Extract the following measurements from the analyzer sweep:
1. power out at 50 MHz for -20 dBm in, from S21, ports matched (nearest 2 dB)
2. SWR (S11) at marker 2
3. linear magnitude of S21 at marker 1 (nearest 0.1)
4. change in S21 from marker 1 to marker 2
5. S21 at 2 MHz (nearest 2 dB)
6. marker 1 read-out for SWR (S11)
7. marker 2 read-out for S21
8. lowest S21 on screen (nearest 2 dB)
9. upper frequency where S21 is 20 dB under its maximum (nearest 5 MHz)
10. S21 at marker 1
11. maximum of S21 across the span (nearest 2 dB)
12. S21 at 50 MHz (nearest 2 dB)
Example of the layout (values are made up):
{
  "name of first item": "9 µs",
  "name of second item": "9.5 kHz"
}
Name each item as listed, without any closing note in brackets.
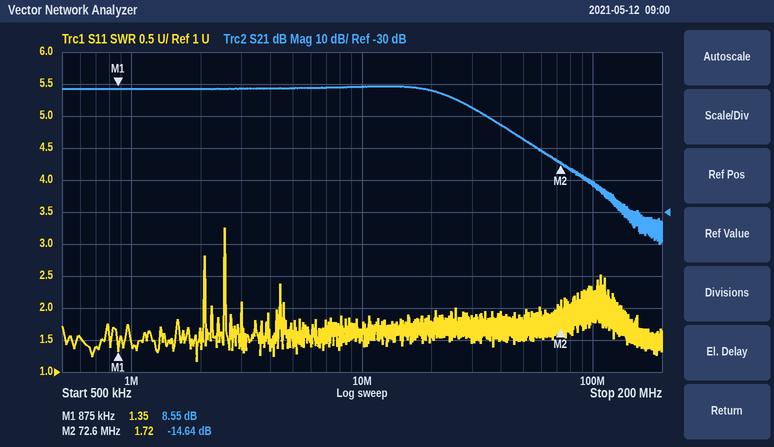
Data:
{
  "power out at 50 MHz for -20 dBm in, from S21, ports matched": "-28 dBm",
  "SWR (S11) at marker 2": "1.72",
  "linear magnitude of S21 at marker 1": "2.7",
  "change in S21 from marker 1 to marker 2": "-23.19 dB",
  "S21 at 2 MHz": "8 dB",
  "marker 1 read-out for SWR": "1.35",
  "marker 2 read-out for S21": "-14.64 dB",
  "lowest S21 on screen": "-40 dB",
  "upper frequency where S21 is 20 dB under its maximum": "60 MHz",
  "S21 at marker 1": "8.55 dB",
  "maximum of S21 across the span": "10 dB",
  "S21 at 50 MHz": "-8 dB"
}
